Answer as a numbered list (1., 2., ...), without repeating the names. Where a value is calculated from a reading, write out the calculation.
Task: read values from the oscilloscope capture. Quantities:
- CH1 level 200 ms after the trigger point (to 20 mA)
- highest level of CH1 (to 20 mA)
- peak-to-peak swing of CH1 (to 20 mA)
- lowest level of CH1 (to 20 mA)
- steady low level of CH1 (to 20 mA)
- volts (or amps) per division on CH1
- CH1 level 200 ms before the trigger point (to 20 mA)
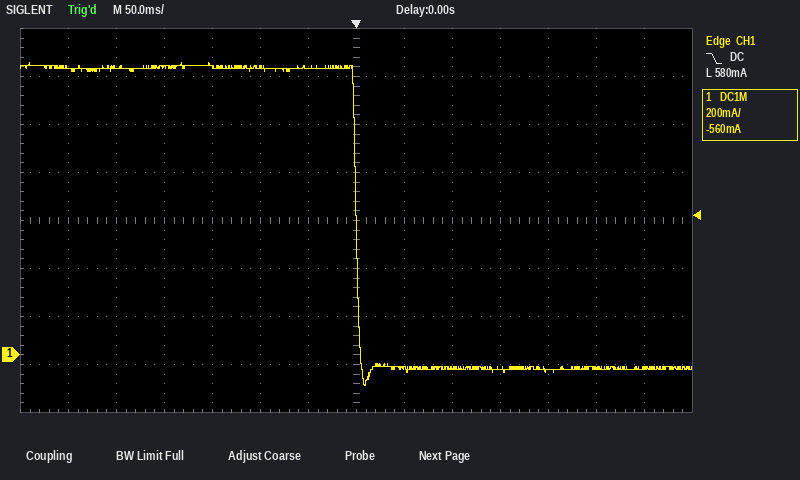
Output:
1. -60 mA
2. 1.22 A
3. 1.22 A − (-120 mA) = 1.34 A
4. -120 mA
5. -60 mA
6. 200 mA
7. 1.20 A
